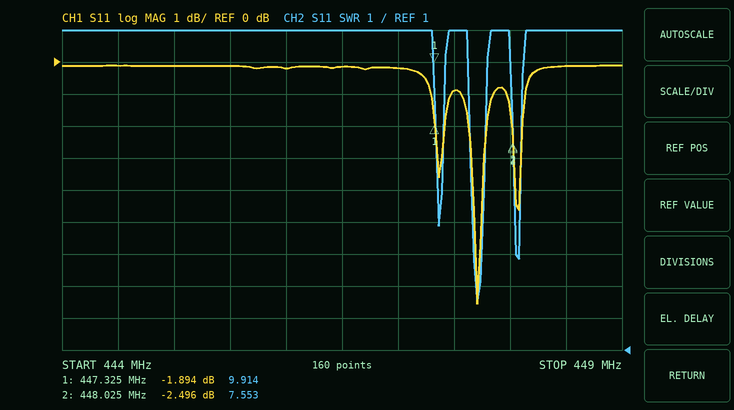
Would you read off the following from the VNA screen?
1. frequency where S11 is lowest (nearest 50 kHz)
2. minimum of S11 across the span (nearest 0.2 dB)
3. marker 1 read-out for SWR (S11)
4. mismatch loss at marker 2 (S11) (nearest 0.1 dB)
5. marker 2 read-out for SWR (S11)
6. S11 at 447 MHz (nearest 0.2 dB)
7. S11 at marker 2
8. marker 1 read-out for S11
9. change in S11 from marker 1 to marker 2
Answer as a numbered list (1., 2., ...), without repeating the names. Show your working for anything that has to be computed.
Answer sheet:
1. 447.70 MHz
2. -7.6 dB
3. 9.914
4. −10 log10(1 − 10^(-2.496/10)) ≈ 3.6 dB
5. 7.553
6. -0.2 dB
7. -2.496 dB
8. -1.894 dB
9. -2.496 − (-1.894) = -0.602 dB
